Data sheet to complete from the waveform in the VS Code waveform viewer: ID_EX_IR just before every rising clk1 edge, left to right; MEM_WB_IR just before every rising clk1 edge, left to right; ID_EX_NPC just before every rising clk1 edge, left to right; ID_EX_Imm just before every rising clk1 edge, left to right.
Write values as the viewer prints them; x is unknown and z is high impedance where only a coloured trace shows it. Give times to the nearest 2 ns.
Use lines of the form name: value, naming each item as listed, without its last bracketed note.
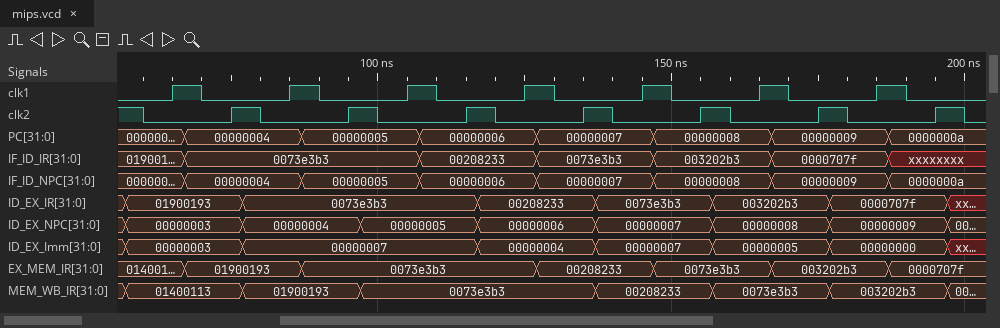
ID_EX_IR just before every rising clk1 edge, left to right: 01900193, 0073e3b3, 0073e3b3, 00208233, 0073e3b3, 003202b3, 0000707f
MEM_WB_IR just before every rising clk1 edge, left to right: 01400113, 01900193, 0073e3b3, 0073e3b3, 00208233, 0073e3b3, 003202b3
ID_EX_NPC just before every rising clk1 edge, left to right: 00000003, 00000004, 00000005, 00000006, 00000007, 00000008, 00000009
ID_EX_Imm just before every rising clk1 edge, left to right: 00000003, 00000007, 00000007, 00000004, 00000007, 00000005, 00000000
